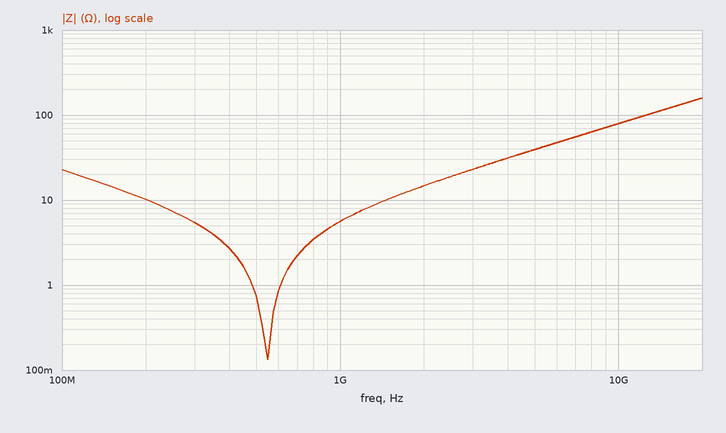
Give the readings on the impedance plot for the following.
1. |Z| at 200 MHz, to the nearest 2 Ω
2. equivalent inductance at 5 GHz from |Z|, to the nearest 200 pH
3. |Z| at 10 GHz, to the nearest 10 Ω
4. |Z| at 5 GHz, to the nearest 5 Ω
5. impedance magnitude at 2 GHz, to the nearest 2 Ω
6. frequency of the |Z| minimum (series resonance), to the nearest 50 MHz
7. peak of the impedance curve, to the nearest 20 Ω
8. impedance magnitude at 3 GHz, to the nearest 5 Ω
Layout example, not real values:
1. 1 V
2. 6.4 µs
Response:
1. 10 Ω
2. 1.2 nH
3. 80 Ω
4. 40 Ω
5. 14 Ω
6. 550 MHz
7. 160 Ω
8. 25 Ω
